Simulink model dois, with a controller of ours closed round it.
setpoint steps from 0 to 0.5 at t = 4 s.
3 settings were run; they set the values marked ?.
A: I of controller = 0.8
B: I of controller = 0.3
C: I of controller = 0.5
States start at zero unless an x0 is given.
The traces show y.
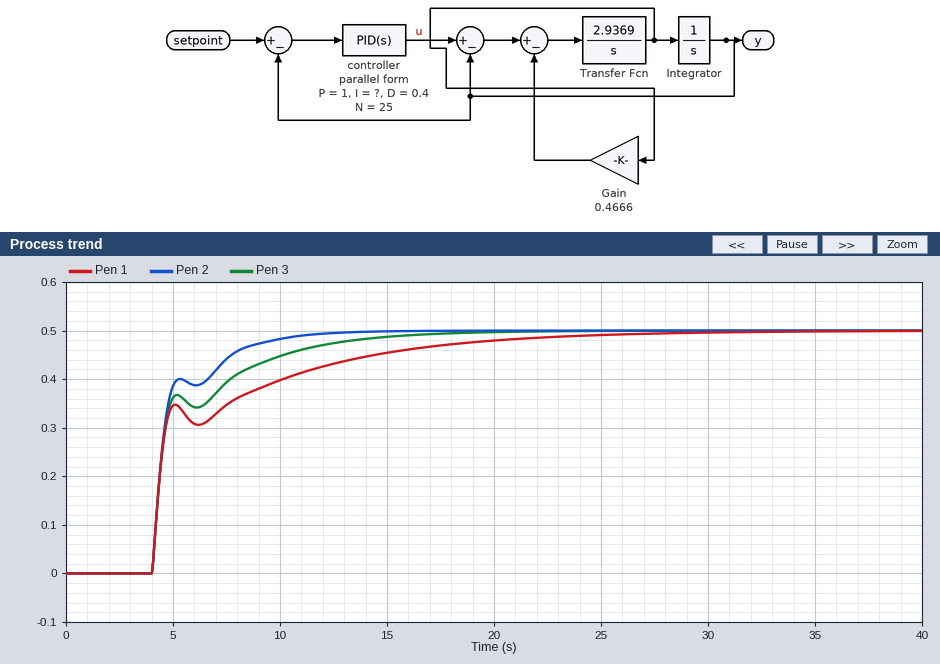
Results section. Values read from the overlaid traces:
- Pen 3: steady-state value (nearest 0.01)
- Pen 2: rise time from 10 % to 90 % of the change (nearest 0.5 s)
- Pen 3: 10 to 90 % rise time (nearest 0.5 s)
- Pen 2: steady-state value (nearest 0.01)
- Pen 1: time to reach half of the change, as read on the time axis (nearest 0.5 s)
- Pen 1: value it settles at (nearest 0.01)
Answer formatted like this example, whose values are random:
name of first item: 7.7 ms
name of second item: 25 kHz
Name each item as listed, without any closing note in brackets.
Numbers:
Pen 3: steady-state value: 0.50
Pen 2: rise time from 10 % to 90 % of the change: 3.5 s
Pen 3: 10 to 90 % rise time: 6.0 s
Pen 2: steady-state value: 0.50
Pen 1: time to reach half of the change, as read on the time axis: 4.5 s
Pen 1: value it settles at: 0.50
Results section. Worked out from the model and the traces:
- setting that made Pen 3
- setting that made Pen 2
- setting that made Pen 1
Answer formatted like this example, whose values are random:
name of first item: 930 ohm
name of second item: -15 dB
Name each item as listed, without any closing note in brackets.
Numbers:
setting that made Pen 3: C
setting that made Pen 2: A
setting that made Pen 1: B
